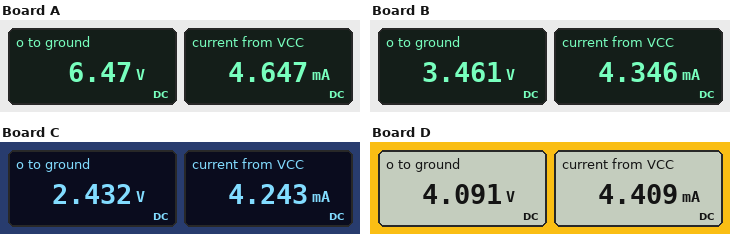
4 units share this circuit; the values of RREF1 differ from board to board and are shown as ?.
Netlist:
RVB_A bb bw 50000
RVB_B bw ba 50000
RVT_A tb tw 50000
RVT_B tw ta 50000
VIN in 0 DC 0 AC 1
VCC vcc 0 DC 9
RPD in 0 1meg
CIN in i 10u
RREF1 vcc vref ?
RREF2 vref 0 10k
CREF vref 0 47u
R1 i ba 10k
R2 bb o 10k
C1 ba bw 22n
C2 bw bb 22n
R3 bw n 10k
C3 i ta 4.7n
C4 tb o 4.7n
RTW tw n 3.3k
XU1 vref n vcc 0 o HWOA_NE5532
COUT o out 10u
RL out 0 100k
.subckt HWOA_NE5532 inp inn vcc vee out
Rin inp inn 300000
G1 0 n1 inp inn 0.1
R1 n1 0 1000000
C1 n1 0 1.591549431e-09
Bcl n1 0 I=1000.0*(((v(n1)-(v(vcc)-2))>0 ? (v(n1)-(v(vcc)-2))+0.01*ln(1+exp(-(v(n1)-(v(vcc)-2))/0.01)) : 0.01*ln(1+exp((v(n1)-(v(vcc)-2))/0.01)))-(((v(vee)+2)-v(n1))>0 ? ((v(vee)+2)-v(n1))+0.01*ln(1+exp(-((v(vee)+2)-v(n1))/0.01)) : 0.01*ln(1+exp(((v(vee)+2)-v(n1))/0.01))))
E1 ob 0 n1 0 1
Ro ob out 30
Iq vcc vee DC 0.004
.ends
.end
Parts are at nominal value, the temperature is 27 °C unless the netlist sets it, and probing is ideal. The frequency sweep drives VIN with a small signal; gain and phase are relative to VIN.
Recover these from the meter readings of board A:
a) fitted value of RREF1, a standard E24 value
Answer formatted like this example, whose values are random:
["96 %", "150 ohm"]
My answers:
["3.9 kΩ"]
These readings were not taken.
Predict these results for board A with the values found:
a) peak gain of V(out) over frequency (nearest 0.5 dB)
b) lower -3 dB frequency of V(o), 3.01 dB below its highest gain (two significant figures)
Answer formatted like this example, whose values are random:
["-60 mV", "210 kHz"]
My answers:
["0 dB", "270 mHz"]
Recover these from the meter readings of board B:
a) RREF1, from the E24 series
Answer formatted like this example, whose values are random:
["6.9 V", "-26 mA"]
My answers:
["16 kΩ"]
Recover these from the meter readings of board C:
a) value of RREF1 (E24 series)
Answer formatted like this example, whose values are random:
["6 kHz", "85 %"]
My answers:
["27 kΩ"]
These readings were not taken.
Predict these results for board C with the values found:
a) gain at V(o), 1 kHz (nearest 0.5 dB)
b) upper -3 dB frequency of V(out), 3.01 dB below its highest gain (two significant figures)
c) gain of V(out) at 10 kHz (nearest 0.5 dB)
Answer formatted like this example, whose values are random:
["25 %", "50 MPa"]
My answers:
["0 dB", "4.8 MHz", "0 dB"]
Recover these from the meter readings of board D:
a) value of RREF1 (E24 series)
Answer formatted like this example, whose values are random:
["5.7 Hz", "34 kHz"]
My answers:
["12 kΩ"]
